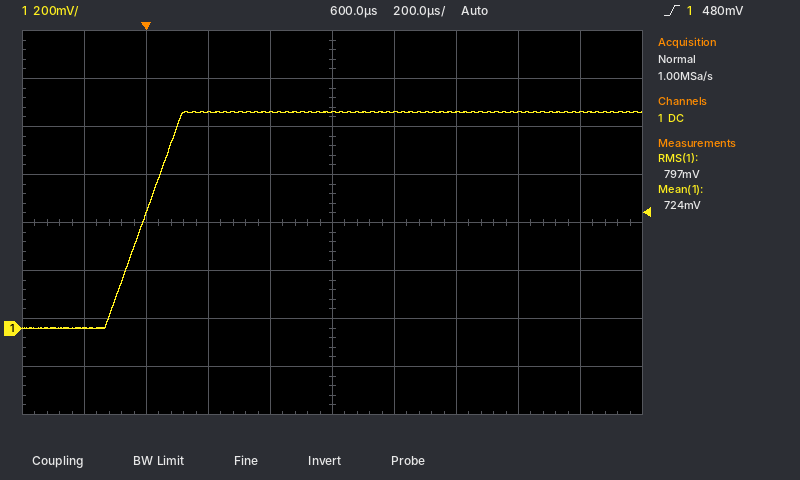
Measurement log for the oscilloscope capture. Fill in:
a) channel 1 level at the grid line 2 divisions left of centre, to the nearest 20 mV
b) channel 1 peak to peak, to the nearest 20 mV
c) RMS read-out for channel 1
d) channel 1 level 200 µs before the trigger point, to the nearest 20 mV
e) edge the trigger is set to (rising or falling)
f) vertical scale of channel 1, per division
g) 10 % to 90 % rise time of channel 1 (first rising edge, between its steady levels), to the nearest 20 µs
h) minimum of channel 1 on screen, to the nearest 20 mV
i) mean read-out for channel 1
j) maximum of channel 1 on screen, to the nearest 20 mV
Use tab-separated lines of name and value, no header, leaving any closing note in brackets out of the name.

channel 1 level at the grid line 2 divisions left of centre, to the nearest 20 mV	900 mV
channel 1 peak to peak, to the nearest 20 mV	900 mV
RMS read-out for channel 1	797 mV
channel 1 level 200 µs before the trigger point, to the nearest 20 mV	0 mV
edge the trigger is set to	rising
vertical scale of channel 1, per division	200 mV
10 % to 90 % rise time of channel 1 (first rising edge, between its steady levels), to the nearest 20 µs	200 µs
minimum of channel 1 on screen, to the nearest 20 mV	0 mV
mean read-out for channel 1	724 mV
maximum of channel 1 on screen, to the nearest 20 mV	900 mV
